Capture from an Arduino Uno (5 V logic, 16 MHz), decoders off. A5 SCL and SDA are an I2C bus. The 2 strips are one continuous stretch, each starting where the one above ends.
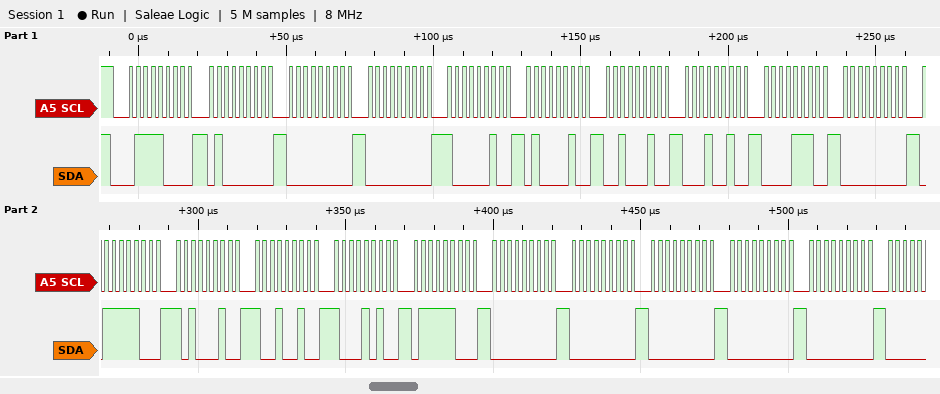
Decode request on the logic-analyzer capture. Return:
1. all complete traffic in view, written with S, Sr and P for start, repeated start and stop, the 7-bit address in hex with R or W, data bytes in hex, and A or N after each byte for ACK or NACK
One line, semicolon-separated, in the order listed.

S 3CW A 40 A 00 A 00 A 82 A 42 A 22 A 12 A 0E A 00 A 7C A A2 A 92 A 8A A 7C A 00 A 00 A 00 A 00 A 00 A
